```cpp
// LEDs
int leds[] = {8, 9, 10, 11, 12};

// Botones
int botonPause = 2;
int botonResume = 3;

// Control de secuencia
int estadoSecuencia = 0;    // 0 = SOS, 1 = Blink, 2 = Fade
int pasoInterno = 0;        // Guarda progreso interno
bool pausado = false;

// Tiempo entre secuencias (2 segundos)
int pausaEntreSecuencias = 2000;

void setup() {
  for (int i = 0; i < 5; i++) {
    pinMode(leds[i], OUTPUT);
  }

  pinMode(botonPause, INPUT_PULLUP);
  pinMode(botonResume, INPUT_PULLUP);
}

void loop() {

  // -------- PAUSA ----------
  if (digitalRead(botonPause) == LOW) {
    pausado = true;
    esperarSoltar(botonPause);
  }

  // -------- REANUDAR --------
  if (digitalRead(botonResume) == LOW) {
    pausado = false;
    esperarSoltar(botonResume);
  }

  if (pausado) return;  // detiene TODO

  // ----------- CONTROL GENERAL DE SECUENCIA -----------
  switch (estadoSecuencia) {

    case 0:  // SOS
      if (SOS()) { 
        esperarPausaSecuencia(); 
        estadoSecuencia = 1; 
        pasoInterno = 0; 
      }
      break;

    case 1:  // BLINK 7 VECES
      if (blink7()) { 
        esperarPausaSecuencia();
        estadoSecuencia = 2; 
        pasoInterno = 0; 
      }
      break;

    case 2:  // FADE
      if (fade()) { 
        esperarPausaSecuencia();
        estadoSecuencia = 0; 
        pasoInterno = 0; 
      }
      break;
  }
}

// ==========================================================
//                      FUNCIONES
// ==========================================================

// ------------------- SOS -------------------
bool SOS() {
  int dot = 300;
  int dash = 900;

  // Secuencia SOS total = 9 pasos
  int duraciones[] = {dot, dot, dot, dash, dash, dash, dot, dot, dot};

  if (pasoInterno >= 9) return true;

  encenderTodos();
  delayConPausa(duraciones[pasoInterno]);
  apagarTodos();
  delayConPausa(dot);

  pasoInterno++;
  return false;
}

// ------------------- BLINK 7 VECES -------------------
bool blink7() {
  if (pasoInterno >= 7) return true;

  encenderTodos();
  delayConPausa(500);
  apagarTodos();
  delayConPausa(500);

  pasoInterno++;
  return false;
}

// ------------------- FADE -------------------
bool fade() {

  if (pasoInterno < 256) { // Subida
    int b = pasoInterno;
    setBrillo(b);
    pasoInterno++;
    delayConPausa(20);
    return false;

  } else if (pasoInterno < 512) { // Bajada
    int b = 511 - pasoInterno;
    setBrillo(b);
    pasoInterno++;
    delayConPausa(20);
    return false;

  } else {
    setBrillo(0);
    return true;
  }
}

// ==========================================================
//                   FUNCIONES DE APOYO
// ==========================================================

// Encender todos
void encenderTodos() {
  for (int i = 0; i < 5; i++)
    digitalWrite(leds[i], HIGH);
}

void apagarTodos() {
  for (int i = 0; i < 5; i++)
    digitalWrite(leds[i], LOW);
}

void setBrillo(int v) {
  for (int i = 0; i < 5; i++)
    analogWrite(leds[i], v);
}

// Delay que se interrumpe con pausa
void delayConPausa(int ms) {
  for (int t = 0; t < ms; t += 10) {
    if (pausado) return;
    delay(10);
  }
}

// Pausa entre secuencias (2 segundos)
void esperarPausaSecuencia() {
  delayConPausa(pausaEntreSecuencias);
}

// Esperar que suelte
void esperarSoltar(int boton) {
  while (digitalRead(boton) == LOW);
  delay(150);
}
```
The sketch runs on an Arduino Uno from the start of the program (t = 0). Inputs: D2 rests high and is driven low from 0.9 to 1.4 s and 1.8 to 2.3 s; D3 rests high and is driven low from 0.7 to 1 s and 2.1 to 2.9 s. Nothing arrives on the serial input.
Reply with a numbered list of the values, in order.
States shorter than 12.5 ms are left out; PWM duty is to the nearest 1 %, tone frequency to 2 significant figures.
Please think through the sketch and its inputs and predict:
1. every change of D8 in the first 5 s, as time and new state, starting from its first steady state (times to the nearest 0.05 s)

1. 0 s high; 0.3 s low; 0.6 s high; 0.9 s low; 3.05 s high; 3.35 s low; 3.65 s high; 4.55 s low; 4.85 s high
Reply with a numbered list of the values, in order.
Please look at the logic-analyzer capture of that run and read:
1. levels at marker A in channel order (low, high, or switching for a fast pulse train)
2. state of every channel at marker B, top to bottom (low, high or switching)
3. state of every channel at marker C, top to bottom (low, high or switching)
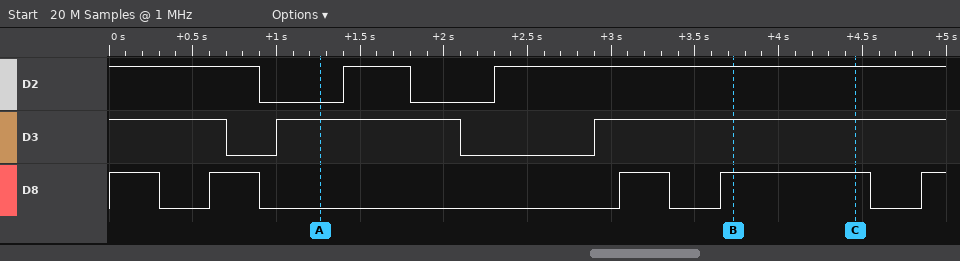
1. D2 low, D3 high, D8 low
2. D2 high, D3 high, D8 high
3. D2 high, D3 high, D8 high
